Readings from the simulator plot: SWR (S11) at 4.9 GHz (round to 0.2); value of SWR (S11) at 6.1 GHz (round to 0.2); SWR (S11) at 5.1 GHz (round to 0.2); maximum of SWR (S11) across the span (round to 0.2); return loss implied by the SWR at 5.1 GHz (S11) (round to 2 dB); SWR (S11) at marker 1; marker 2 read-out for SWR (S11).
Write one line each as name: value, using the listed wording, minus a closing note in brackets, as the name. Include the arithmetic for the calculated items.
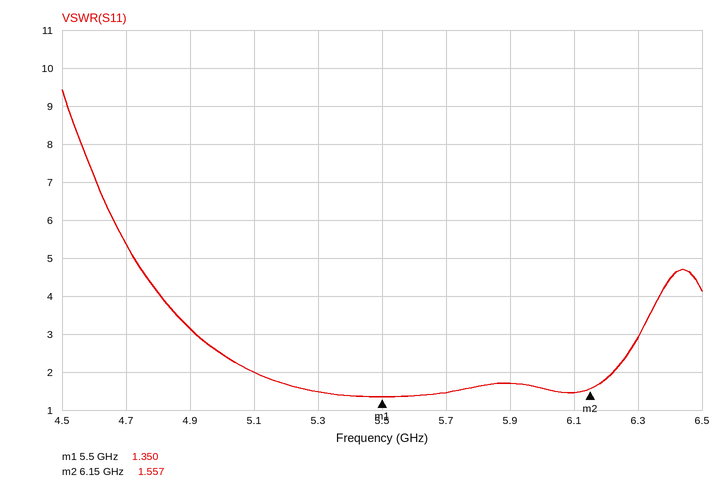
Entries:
SWR (S11) at 4.9 GHz: 3.2
value of SWR (S11) at 6.1 GHz: 1.4
SWR (S11) at 5.1 GHz: 2.0
maximum of SWR (S11) across the span: 9.4
return loss implied by the SWR at 5.1 GHz (S11): −20 log10((2 − 1)/(2 + 1)) ≈ 10 dB
SWR (S11) at marker 1: 1.350
marker 2 read-out for SWR: 1.557
